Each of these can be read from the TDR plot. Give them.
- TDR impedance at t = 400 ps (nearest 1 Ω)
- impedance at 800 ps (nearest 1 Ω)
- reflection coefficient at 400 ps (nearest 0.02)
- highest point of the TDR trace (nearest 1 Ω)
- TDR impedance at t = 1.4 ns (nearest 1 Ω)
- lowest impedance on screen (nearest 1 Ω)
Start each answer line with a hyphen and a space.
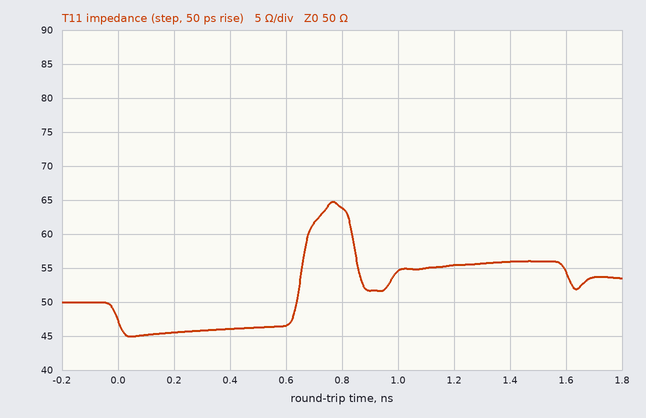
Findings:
- 46 Ω
- 64 Ω
- -0.04
- 65 Ω
- 56 Ω
- 45 Ω
